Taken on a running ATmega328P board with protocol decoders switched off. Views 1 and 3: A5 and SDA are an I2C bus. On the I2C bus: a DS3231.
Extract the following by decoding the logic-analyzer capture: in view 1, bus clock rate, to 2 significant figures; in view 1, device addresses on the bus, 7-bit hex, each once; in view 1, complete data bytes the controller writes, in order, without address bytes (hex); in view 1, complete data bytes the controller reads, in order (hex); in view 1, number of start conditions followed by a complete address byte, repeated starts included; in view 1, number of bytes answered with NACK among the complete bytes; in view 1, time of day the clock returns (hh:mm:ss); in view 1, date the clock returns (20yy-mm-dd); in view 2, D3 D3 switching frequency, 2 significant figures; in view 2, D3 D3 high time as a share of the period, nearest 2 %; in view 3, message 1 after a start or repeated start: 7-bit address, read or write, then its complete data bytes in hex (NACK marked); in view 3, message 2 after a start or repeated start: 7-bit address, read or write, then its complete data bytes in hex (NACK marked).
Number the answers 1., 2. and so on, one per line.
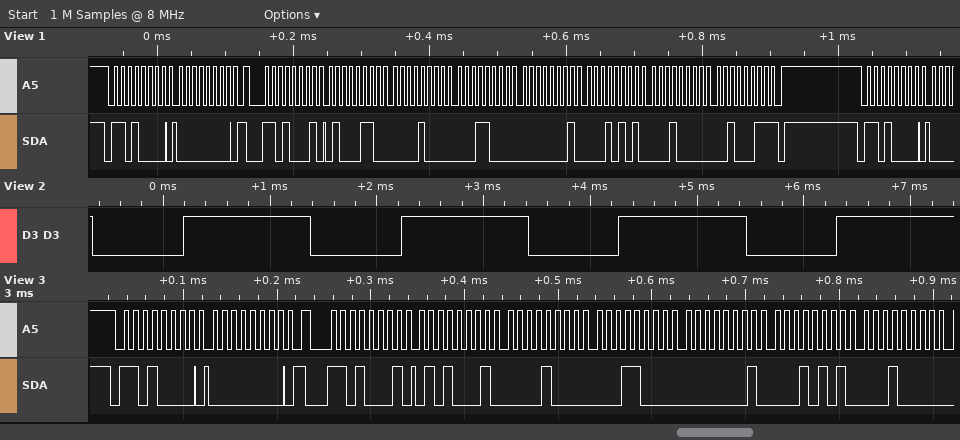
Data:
1. 100 kHz
2. 0x68
3. 00
4. 46 08 18 01 15 10 23
5. 3
6. 1
7. 18:08:46
8. 2023-10-15
9. 490 Hz
10. 58 %
11. 0x68 write: 00
12. 0x68 read: 51 08 18 01 15 10
